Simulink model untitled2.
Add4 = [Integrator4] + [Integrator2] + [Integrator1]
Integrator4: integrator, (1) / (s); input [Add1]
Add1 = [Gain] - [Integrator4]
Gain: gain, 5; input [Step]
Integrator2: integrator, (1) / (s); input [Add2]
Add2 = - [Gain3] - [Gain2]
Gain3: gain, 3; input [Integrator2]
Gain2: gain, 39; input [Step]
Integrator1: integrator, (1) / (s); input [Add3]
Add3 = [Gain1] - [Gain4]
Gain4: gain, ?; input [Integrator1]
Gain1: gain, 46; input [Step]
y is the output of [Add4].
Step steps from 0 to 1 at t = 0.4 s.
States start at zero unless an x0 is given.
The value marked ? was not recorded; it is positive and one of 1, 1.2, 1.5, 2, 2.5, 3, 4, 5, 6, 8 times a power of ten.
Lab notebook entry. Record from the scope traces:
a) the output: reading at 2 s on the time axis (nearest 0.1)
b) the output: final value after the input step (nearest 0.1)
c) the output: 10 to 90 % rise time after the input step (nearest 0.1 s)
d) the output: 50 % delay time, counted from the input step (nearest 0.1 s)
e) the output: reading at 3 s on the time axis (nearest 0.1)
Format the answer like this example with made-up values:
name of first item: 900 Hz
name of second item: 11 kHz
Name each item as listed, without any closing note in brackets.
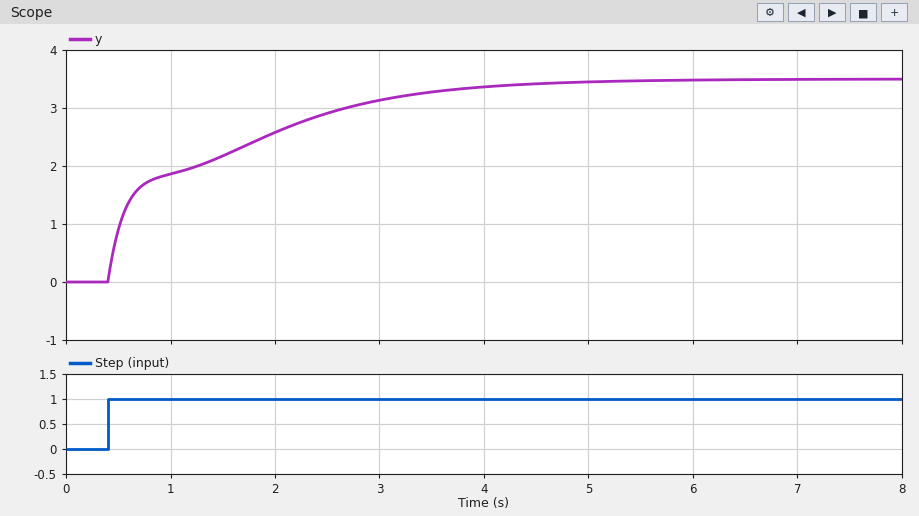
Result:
the output: reading at 2 s on the time axis: 2.6
the output: final value after the input step: 3.5
the output: 10 to 90 % rise time after the input step: 2.6 s
the output: 50 % delay time, counted from the input step: 0.4 s
the output: reading at 3 s on the time axis: 3.1
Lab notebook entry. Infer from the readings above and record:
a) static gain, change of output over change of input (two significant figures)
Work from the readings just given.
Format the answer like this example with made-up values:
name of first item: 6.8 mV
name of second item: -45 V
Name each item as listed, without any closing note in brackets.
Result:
static gain, change of output over change of input: 3.5
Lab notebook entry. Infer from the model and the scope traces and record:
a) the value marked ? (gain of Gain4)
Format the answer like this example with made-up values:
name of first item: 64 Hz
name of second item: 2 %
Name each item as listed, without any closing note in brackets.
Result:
the value marked ?: 4
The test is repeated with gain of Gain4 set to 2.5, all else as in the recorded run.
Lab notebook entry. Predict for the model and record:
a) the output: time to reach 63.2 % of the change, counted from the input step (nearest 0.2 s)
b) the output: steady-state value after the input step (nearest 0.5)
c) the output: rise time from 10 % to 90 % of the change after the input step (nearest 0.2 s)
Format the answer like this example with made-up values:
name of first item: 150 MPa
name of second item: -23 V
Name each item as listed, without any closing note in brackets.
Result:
the output: time to reach 63.2 % of the change, counted from the input step: 0.8 s
the output: steady-state value after the input step: 10.5
the output: rise time from 10 % to 90 % of the change after the input step: 1.6 s
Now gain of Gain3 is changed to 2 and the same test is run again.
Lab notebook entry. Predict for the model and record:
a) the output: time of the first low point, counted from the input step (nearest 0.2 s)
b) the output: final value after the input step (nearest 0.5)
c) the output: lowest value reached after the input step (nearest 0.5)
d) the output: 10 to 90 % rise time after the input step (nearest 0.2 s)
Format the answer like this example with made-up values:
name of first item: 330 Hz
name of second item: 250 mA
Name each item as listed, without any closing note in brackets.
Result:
the output: time of the first low point, counted from the input step: 2.0 s
the output: final value after the input step: -3.0
the output: lowest value reached after the input step: -3.5
the output: 10 to 90 % rise time after the input step: 0.6 s
